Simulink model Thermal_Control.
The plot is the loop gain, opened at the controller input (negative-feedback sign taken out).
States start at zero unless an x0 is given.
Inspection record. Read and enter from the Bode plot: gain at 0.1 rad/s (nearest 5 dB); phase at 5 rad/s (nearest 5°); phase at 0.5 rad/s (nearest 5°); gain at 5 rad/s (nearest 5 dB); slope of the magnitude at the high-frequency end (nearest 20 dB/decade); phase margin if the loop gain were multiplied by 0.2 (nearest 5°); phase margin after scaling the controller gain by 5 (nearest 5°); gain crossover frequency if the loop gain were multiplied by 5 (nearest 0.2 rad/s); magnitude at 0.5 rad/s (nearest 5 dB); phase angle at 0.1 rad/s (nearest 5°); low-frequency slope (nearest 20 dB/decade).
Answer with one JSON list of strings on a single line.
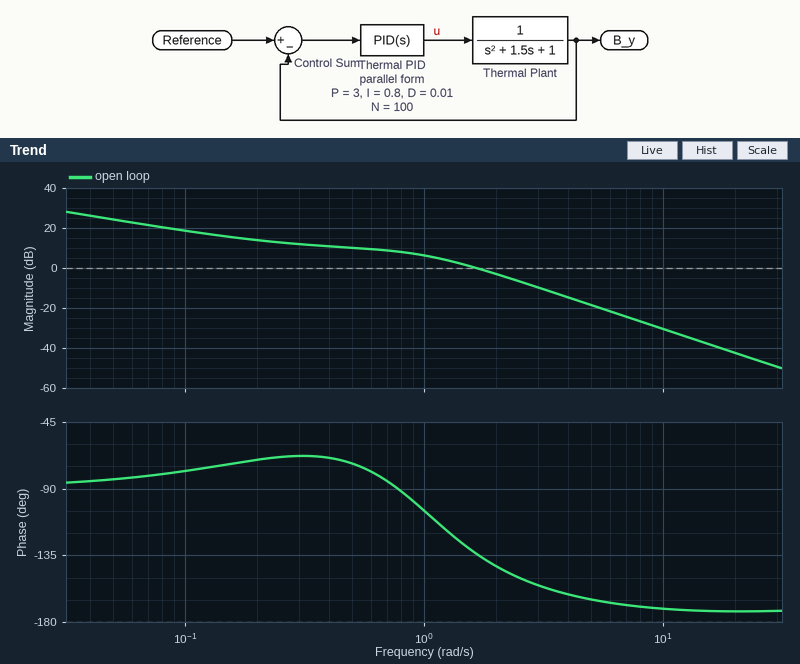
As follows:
["20 dB", "-165°", "-75°", "-20 dB", "-40 dB/decade", "110°", "20°", "3.8 rad/s", "10 dB", "-80°", "-20 dB/decade"]
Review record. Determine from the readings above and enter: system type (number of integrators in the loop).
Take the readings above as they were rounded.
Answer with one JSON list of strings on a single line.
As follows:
["1"]
